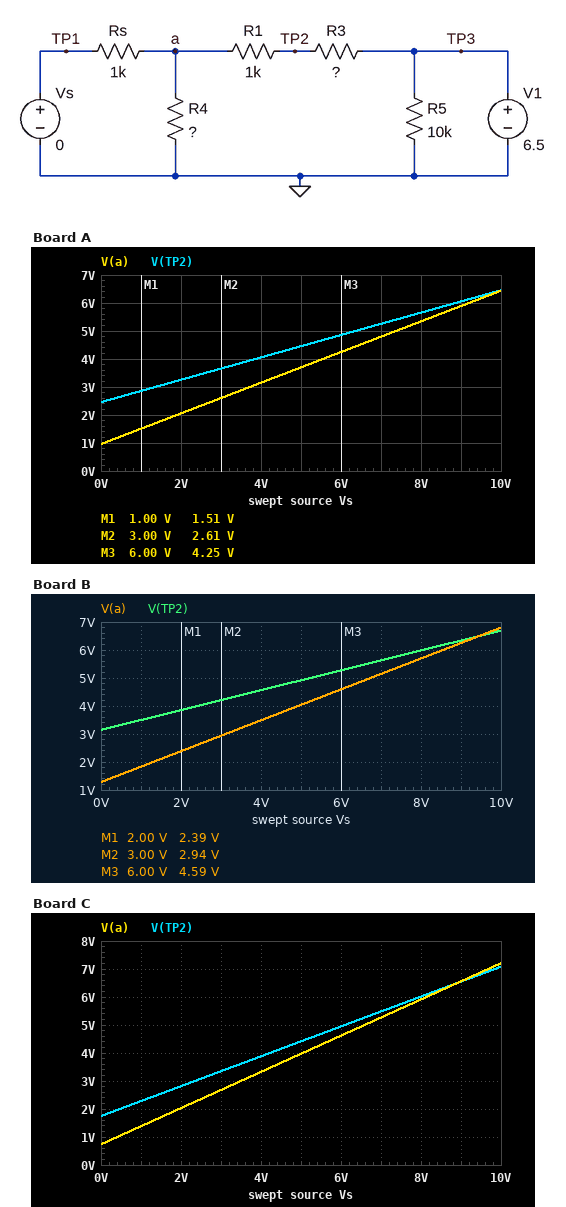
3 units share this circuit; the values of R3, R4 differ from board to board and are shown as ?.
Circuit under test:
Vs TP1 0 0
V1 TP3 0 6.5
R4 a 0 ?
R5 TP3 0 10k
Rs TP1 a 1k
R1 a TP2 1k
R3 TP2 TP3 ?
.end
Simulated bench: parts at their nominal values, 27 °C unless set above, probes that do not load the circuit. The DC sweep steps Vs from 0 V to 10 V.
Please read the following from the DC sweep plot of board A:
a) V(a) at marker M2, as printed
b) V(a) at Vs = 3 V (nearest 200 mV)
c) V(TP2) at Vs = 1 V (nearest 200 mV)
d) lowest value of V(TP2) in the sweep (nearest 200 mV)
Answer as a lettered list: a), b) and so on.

a) 2.61 V
b) 2.6 V
c) 2.8 V
d) 2.4 V
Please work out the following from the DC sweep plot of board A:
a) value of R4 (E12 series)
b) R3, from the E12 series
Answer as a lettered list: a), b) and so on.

a) 1.8 kΩ
b) 2.7 kΩ
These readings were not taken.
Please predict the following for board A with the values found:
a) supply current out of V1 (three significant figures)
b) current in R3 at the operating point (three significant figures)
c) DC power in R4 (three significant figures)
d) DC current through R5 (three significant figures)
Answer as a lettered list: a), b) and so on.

a) 2.15 mA
b) 1.50 mA
c) 514 µW
d) 650 µA
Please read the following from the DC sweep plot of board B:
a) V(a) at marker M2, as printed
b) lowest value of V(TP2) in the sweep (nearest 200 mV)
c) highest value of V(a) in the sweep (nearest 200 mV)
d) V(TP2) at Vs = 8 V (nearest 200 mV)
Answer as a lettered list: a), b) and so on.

a) 2.94 V
b) 3.2 V
c) 6.8 V
d) 6.0 V
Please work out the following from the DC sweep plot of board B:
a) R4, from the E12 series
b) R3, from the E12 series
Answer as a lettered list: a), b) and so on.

a) 2.2 kΩ
b) 1.8 kΩ
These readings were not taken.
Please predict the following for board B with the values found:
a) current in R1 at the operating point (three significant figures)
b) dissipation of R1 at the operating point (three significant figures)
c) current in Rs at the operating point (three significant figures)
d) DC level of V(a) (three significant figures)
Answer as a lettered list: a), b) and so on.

a) 1.86 mA
b) 3.47 mW
c) 1.28 mA
d) 1.28 V
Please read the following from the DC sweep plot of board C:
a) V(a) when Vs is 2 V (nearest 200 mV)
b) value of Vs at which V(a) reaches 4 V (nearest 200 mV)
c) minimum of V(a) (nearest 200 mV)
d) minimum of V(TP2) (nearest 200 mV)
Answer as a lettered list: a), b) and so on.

a) 2.0 V
b) 5.0 V
c) 800 mV
d) 1.8 V
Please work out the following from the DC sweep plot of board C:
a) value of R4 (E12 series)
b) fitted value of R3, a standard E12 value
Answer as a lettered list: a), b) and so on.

a) 2.7 kΩ
b) 4.7 kΩ
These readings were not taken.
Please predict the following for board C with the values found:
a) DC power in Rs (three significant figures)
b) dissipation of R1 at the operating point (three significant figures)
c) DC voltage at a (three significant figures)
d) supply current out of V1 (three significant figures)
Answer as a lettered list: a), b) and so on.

a) 544 µW
b) 1.02 mW
c) 738 mV
d) 1.66 mA
